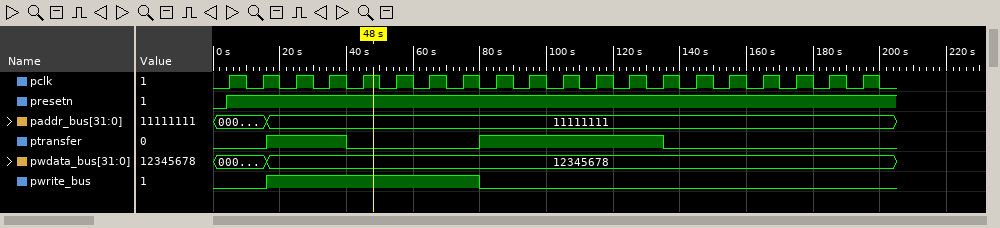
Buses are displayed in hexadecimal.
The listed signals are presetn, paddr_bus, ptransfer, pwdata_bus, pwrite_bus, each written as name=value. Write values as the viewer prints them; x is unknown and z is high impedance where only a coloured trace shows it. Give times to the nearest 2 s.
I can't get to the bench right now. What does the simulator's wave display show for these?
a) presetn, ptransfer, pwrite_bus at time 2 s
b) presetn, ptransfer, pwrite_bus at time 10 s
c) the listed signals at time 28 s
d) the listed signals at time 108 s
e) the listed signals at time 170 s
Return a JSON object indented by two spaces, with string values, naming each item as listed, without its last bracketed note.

{
  "presetn, ptransfer, pwrite_bus at time 2 s": "presetn=0, ptransfer=0, pwrite_bus=0",
  "presetn, ptransfer, pwrite_bus at time 10 s": "presetn=1, ptransfer=0, pwrite_bus=0",
  "the listed signals at time 28 s": "presetn=1, paddr_bus=11111111, ptransfer=1, pwdata_bus=12345678, pwrite_bus=1",
  "the listed signals at time 108 s": "presetn=1, paddr_bus=11111111, ptransfer=1, pwdata_bus=12345678, pwrite_bus=0",
  "the listed signals at time 170 s": "presetn=1, paddr_bus=11111111, ptransfer=0, pwdata_bus=12345678, pwrite_bus=0"
}
